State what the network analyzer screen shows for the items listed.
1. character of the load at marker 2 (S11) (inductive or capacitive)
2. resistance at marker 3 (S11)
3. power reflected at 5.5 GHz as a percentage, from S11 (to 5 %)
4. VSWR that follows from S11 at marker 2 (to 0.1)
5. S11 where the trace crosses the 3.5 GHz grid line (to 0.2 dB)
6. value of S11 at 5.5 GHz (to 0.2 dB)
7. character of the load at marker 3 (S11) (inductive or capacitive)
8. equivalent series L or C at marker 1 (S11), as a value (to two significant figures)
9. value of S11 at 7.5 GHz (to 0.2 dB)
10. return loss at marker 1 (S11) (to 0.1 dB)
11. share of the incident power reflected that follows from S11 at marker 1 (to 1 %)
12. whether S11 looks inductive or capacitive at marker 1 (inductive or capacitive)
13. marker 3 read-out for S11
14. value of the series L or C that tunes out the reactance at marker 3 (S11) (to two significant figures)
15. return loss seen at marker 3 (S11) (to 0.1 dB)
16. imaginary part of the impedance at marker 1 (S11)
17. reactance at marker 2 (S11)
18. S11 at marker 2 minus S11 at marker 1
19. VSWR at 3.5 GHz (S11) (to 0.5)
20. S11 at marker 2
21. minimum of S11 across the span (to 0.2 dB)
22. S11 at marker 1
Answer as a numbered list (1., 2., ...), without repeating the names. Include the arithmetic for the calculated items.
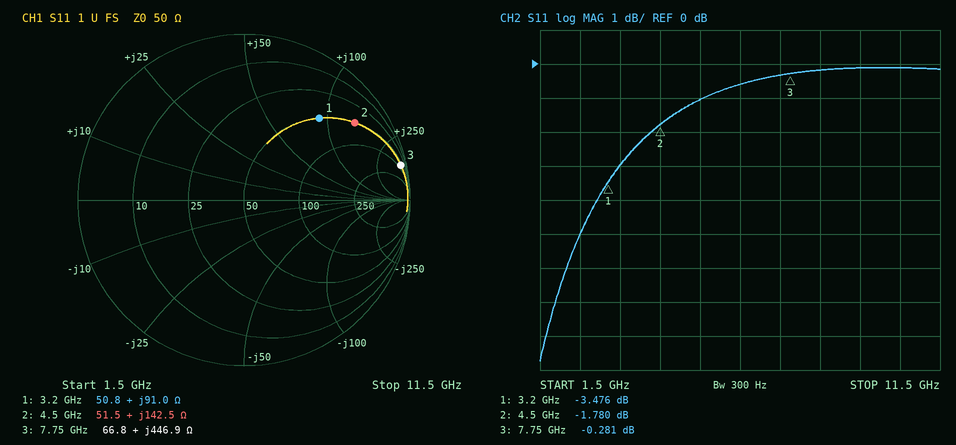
1. inductive
2. 66.8 Ω
3. 10^(-1/10) ≈ 79.4 %, so 80 % to the nearest 5 %
4. (1 + 0.8147)/(1 − 0.8147) ≈ 9.8
5. -3.0 dB
6. -1.0 dB
7. inductive
8. L = 91 Ω/(2π × 3.2 GHz) ≈ 4.5 nH
9. -0.4 dB
10. 3.5 dB
11. 10^(-3.476/10) ≈ 45 %
12. inductive
13. -0.281 dB
14. C = 1/(2π × 7.75 GHz × 446.9 Ω) ≈ 46 fF
15. 0.3 dB
16. +91.0 Ω
17. +142.5 Ω
18. -1.78 − (-3.476) = 1.696 dB
19. |Γ| = 10^(-3/20) = 0.7079; VSWR = (1 + 0.7079)/(1 − 0.7079) ≈ 5.85, so 6.0 to the nearest 0.5
20. -1.780 dB
21. -8.8 dB
22. -3.476 dB
